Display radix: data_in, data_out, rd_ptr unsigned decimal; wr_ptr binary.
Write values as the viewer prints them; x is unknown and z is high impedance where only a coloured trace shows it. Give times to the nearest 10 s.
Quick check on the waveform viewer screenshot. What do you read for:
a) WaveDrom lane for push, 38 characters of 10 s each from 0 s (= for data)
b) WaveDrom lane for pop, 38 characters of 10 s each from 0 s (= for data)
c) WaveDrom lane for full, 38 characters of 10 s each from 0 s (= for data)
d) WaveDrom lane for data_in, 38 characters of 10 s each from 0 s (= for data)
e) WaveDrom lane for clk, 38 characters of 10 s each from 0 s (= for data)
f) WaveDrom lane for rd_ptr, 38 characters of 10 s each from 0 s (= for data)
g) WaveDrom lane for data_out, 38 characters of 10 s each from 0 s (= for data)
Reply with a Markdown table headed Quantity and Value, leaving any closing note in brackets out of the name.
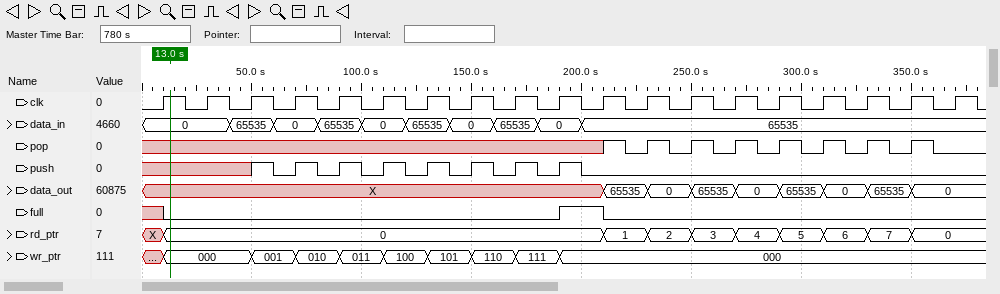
| Quantity | Value |
|---|---|
| WaveDrom lane for push, 38 characters of 10 s each from 0 s | {name: 'push', wave: 'x....1010101010101010.................'} |
| WaveDrom lane for pop, 38 characters of 10 s each from 0 s | {name: 'pop', wave: 'x....................1010101010101010.'} |
| WaveDrom lane for full, 38 characters of 10 s each from 0 s | {name: 'full', wave: 'x0.................1.0................'} |
| WaveDrom lane for data_in, 38 characters of 10 s each from 0 s | {name: 'data_in', wave: '=...=.=.=.=.=.=.=.=.=.................', data: '0 65535 0 65535 0 65535 0 65535 0 65535'} |
| WaveDrom lane for clk, 38 characters of 10 s each from 0 s | {name: 'clk', wave: '01010101010101010101010101010101010101'} |
| WaveDrom lane for rd_ptr, 38 characters of 10 s each from 0 s | {name: 'rd_ptr', wave: 'x=...................=.=.=.=.=.=.=.=..', data: '0 1 2 3 4 5 6 7 0'} |
| WaveDrom lane for data_out, 38 characters of 10 s each from 0 s | {name: 'data_out', wave: 'x....................=.=.=.=.=.=.=.=..', data: '65535 0 65535 0 65535 0 65535 0'} |
